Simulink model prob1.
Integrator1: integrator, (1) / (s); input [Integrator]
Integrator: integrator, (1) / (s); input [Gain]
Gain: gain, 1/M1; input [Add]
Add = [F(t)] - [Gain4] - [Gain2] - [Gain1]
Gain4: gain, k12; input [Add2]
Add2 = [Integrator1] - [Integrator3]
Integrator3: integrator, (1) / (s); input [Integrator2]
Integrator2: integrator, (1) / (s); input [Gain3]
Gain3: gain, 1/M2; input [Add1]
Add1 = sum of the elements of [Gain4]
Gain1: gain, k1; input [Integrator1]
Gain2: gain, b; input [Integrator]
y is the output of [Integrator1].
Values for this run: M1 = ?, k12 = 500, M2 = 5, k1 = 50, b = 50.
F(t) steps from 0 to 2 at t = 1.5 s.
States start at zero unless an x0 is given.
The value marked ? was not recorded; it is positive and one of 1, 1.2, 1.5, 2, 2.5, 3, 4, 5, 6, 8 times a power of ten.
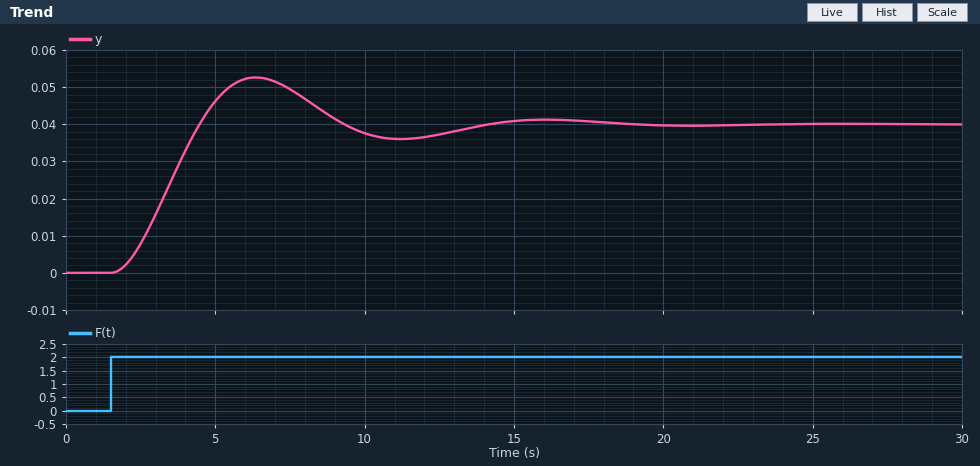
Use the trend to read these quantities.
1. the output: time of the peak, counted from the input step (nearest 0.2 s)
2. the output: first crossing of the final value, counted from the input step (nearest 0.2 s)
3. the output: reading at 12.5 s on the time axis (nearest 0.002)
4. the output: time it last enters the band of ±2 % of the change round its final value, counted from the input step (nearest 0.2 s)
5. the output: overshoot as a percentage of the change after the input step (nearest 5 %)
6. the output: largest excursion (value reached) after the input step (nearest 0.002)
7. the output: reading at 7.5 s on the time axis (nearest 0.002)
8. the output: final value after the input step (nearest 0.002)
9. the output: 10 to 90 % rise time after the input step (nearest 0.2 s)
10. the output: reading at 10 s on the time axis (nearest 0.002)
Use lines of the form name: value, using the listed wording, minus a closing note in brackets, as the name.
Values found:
the output: time of the peak, counted from the input step: 4.8 s
the output: first crossing of the final value, counted from the input step: 3.0 s
the output: reading at 12.5 s on the time axis: 0.038
the output: time it last enters the band of ±2 % of the change round its final value, counted from the input step: 16.0 s
the output: overshoot as a percentage of the change after the input step: 30 %
the output: largest excursion (value reached) after the input step: 0.052
the output: reading at 7.5 s on the time axis: 0.050
the output: final value after the input step: 0.040
the output: 10 to 90 % rise time after the input step: 2.0 s
the output: reading at 10 s on the time axis: 0.038
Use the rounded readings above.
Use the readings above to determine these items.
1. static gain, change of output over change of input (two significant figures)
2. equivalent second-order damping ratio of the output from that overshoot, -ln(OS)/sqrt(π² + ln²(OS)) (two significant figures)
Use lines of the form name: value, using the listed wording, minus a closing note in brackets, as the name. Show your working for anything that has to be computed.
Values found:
static gain, change of output over change of input: (0.04 - 0) / (2 - 0) = 0.020
equivalent second-order damping ratio of the output from that overshoot, -ln(OS)/sqrt(π² + ln²(OS)): ln(0.3) = -1.204; 1.204 / sqrt(9.870 + 1.450) = 0.36
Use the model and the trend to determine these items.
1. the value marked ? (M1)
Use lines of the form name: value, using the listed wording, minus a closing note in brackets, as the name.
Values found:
the value marked ?: 100
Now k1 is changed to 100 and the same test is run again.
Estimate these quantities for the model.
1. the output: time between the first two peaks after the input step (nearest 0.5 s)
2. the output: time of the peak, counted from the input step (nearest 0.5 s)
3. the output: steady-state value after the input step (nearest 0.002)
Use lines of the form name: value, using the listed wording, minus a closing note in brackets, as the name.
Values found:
the output: time between the first two peaks after the input step: 6.5 s
the output: time of the peak, counted from the input step: 3.5 s
the output: steady-state value after the input step: 0.020
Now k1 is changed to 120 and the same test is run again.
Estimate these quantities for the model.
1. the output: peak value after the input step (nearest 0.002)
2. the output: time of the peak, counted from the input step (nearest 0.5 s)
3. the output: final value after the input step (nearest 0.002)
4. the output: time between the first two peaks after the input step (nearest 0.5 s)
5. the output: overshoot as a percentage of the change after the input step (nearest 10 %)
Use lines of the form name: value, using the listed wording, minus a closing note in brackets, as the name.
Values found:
the output: peak value after the input step: 0.024
the output: time of the peak, counted from the input step: 3.0 s
the output: final value after the input step: 0.016
the output: time between the first two peaks after the input step: 6.0 s
the output: overshoot as a percentage of the change after the input step: 50 %
